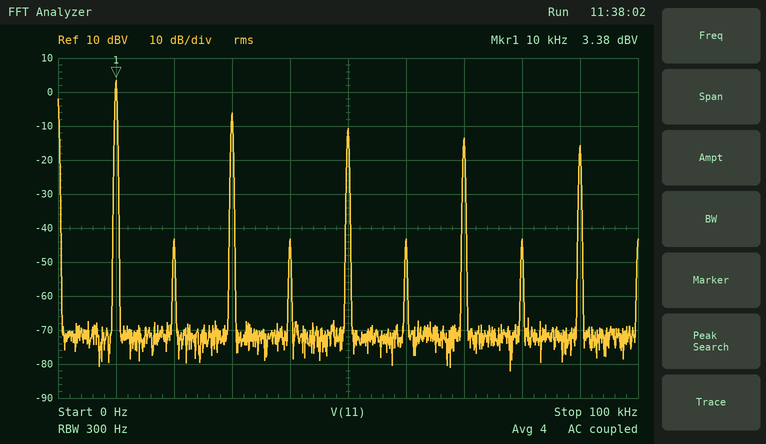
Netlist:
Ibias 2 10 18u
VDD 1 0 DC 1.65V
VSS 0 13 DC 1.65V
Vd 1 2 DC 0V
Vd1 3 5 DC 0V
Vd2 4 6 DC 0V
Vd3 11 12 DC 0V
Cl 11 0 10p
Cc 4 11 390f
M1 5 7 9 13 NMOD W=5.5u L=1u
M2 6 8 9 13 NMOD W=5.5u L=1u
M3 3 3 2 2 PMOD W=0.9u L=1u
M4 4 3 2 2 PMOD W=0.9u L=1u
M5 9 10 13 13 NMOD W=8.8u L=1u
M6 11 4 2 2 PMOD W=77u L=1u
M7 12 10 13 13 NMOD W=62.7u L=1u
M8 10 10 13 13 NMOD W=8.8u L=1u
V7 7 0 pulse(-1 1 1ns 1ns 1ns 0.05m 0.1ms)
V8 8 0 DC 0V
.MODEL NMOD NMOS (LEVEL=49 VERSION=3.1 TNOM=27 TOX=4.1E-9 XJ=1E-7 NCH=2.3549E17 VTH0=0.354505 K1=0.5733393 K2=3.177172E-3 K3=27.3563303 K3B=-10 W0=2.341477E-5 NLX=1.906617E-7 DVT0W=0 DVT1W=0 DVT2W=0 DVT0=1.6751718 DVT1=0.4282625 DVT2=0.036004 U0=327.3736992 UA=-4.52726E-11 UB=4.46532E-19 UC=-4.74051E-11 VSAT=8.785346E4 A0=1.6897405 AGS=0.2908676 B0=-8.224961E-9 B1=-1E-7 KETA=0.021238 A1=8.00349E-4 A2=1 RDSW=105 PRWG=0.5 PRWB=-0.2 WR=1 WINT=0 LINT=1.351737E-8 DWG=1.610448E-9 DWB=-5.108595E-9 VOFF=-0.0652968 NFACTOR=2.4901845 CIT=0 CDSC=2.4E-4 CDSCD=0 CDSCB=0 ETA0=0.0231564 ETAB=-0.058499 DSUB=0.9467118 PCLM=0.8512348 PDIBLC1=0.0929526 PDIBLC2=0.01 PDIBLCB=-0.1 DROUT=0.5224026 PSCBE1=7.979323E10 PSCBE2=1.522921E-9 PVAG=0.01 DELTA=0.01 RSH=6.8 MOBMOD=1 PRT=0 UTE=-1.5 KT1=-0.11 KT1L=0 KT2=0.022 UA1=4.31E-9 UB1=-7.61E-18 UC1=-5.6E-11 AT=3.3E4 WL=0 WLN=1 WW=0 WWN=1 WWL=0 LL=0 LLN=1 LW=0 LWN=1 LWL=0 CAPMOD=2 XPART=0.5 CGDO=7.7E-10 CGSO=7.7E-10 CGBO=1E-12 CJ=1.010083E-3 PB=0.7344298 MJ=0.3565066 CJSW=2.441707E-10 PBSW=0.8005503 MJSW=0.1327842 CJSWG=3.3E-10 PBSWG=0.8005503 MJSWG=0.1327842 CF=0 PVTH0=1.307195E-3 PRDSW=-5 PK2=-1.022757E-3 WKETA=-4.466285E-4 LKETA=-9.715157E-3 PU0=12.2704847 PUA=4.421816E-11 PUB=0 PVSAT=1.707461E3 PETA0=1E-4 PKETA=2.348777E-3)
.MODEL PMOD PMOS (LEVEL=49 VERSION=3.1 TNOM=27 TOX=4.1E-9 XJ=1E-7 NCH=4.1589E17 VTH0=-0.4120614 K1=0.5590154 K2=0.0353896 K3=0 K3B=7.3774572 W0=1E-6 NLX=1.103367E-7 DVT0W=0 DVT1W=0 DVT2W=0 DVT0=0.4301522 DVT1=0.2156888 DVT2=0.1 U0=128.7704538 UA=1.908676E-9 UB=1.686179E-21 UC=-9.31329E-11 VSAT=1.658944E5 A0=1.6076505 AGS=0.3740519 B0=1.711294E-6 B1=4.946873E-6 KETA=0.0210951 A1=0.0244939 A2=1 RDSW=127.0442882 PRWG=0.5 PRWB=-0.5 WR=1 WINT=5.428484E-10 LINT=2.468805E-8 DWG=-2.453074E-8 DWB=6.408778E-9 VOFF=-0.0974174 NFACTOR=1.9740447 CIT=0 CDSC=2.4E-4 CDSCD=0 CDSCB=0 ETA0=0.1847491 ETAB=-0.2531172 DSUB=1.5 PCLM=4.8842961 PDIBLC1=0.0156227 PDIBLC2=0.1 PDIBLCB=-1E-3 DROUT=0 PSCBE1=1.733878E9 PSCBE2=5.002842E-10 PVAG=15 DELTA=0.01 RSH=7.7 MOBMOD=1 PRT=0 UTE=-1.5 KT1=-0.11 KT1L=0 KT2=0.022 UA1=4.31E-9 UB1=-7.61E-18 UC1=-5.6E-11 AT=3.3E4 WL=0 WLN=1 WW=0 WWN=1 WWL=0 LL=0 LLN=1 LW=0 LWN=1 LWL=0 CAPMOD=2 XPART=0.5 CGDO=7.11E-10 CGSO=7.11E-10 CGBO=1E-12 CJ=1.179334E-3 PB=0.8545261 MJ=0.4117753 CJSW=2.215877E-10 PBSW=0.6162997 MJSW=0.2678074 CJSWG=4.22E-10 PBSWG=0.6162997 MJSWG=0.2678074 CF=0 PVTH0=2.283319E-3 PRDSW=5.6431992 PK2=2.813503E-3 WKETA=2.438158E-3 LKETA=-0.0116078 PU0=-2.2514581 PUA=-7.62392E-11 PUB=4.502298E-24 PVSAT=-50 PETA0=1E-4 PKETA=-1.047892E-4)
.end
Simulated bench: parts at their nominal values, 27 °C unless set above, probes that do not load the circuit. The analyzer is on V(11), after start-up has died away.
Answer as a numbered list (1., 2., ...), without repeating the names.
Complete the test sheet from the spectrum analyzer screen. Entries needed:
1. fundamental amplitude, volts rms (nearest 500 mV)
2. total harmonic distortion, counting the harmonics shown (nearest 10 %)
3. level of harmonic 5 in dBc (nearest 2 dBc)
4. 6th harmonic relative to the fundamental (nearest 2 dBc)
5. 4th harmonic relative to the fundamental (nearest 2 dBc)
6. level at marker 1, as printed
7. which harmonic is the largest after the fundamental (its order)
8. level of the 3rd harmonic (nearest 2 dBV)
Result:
1. 1.5 V
2. 40 %
3. -14 dBc
4. -46 dBc
5. -46 dBc
6. 3.38 dBV
7. 3
8. -6 dBV
